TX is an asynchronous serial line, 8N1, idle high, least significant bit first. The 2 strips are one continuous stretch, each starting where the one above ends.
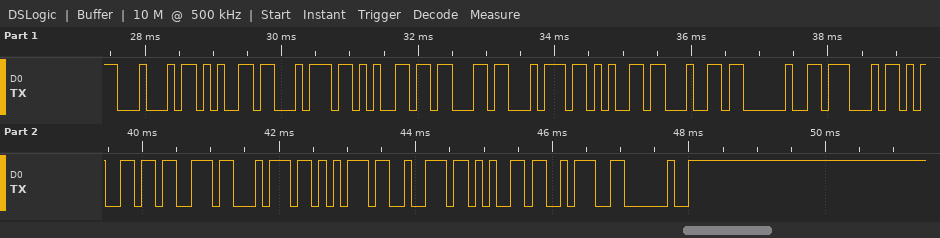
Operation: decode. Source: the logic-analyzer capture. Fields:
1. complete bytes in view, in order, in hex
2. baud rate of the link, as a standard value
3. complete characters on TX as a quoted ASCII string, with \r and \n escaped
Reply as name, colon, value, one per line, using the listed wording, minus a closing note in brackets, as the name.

complete bytes in view, in order, in hex: 0x44 0x65 0x74 0x65 0x63 0x74 0x65 0x64 0x20 0x47 0x65 0x73 0x74 0x75 0x72 0x65 0x3A 0x20
baud rate of the link, as a standard value: 9600 baud
complete characters on TX as a quoted ASCII string, with \r and \n escaped: "Detected Gesture: "
